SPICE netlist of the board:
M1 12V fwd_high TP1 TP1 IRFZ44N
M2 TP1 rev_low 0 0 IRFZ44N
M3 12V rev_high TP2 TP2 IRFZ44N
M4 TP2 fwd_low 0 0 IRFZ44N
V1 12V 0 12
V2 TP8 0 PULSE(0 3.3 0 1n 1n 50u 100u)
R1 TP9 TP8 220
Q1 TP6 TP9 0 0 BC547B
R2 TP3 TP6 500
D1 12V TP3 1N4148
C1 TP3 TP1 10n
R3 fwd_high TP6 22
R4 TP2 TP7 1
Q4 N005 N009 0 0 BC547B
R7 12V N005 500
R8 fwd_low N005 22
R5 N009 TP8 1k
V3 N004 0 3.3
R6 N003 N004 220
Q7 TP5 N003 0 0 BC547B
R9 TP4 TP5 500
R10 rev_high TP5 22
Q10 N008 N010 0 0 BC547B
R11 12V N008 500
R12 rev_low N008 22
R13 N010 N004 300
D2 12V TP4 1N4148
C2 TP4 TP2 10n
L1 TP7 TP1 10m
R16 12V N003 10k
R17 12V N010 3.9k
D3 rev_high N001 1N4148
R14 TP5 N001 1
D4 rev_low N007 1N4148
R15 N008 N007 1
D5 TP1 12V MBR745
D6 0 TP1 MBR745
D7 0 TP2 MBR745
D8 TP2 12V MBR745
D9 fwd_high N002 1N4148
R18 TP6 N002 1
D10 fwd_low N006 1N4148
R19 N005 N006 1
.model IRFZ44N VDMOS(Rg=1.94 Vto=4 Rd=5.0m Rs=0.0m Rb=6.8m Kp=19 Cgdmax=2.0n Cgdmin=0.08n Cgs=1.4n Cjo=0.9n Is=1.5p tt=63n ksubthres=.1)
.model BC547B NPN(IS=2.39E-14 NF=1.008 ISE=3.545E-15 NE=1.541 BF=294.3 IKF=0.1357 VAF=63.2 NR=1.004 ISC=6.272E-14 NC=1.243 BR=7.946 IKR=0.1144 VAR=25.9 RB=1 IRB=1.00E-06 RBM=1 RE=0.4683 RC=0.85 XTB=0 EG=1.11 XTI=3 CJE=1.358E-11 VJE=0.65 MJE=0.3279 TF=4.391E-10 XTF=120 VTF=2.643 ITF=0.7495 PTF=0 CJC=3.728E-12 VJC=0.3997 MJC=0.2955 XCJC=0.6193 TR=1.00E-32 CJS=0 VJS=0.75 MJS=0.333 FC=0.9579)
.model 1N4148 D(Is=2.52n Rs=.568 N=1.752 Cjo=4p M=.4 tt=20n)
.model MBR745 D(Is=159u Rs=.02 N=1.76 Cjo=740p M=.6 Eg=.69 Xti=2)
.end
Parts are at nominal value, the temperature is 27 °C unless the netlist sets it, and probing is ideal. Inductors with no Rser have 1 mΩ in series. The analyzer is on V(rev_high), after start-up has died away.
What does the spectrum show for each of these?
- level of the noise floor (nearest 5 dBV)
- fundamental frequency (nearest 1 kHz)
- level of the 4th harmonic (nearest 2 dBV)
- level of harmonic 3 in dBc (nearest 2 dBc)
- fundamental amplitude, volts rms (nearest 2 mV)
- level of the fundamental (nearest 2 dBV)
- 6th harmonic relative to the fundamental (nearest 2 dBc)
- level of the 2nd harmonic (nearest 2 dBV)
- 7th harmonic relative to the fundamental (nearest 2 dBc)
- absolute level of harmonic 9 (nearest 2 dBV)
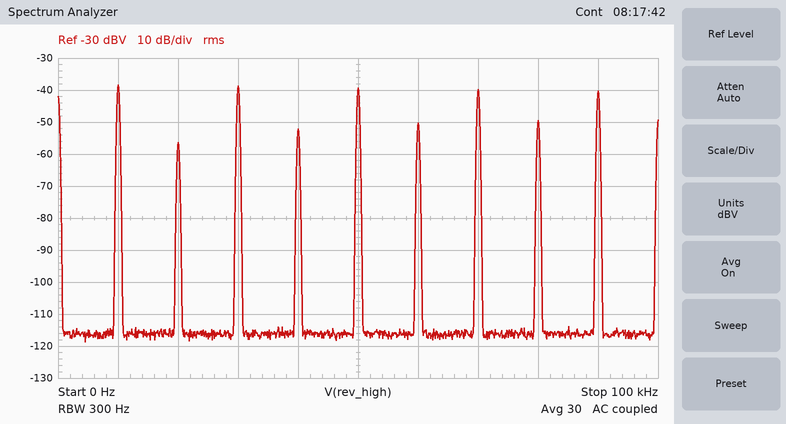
-115 dBV
10 kHz
-52 dBV
0 dBc
12 mV
-38 dBV
-12 dBc
-56 dBV
-2 dBc
-40 dBV
